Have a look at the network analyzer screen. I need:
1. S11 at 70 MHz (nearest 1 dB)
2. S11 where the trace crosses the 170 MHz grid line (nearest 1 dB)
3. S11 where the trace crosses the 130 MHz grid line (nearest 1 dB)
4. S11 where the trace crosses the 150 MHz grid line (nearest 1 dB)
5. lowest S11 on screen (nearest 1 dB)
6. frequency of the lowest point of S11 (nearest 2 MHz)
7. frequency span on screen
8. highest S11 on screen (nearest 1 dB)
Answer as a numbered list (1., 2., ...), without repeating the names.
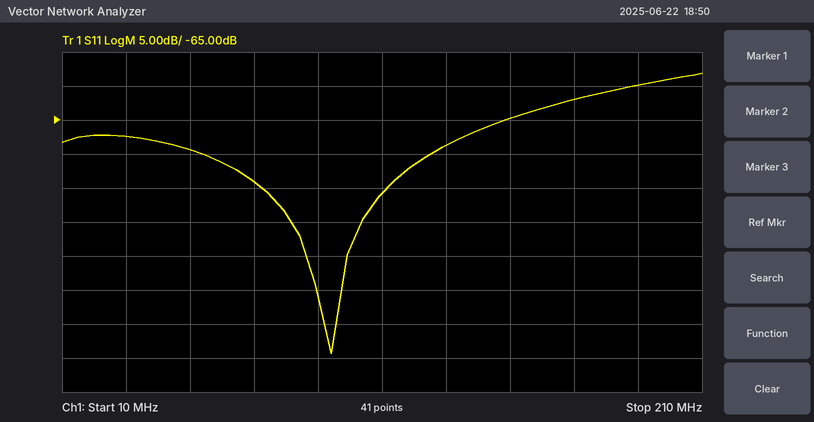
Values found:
1. -74 dB
2. -62 dB
3. -69 dB
4. -65 dB
5. -99 dB
6. 94 MHz
7. 200 MHz
8. -58 dB
